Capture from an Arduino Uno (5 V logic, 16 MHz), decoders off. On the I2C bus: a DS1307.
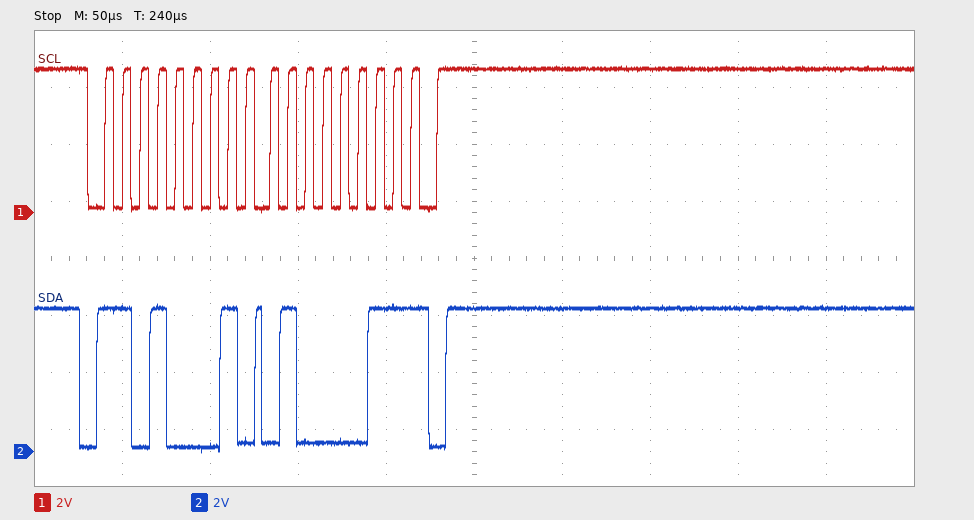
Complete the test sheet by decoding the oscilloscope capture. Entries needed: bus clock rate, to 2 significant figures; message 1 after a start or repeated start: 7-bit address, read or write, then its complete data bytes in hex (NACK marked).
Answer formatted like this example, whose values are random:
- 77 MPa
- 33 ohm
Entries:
- 100 kHz
- 0x68 read: 43 NACK
